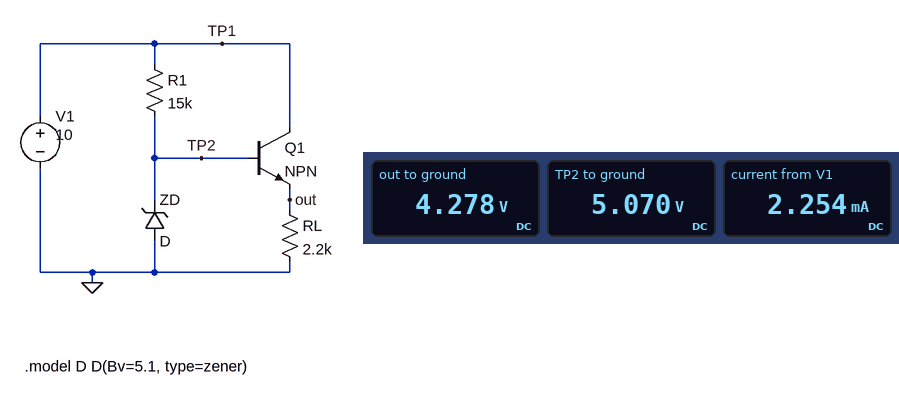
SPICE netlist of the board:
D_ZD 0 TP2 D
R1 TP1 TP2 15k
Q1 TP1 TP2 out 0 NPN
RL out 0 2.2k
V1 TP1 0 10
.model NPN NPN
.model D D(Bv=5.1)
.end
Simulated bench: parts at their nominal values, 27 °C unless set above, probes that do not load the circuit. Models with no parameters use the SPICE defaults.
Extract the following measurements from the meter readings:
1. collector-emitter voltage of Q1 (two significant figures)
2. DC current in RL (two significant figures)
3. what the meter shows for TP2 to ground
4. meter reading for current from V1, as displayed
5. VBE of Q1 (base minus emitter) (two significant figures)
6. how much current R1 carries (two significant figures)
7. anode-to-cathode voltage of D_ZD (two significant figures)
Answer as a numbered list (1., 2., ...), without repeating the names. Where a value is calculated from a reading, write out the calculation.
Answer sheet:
1. 10 V - 4.278 V = 5.7 V
2. (4.278 V) / 2.2 kΩ = 1.9 mA
3. 5.070 V
4. 2.254 mA
5. 5.07 V - 4.278 V = 790 mV
6. (10 V - 5.07 V) / 15 kΩ = 330 µA
7. 0 V - 5.07 V = -5.1 V
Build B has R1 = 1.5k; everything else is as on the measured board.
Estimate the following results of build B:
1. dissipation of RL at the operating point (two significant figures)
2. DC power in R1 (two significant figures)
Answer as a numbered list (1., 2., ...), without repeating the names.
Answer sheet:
1. 8.6 mW
2. 16 mW
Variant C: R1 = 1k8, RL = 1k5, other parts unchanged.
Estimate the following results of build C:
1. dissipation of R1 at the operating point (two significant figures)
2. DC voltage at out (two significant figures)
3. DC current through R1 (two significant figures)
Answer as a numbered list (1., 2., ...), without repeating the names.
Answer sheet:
1. 13 mW
2. 4.3 V
3. 2.7 mA
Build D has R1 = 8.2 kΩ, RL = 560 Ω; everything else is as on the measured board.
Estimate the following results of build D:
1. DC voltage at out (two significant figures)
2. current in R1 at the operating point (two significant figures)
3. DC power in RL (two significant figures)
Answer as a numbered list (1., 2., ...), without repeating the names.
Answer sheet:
1. 4.3 V
2. 600 µA
3. 32 mW
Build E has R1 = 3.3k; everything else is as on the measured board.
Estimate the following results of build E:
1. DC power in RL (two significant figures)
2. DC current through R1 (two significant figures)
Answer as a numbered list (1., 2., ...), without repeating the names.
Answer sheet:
1. 8.5 mW
2. 1.5 mA
